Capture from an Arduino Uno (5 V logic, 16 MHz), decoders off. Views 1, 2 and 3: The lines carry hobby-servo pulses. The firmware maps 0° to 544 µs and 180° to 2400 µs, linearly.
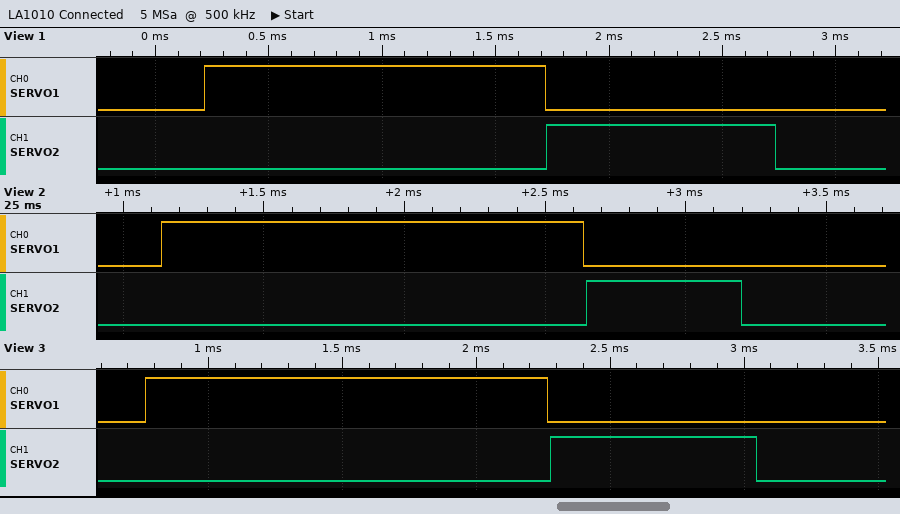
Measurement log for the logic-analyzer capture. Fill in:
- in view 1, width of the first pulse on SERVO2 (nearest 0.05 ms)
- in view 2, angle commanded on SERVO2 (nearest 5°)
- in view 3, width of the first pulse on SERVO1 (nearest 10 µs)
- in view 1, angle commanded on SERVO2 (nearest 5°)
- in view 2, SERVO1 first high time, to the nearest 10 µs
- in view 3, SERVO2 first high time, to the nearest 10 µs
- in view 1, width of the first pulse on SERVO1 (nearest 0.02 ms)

1.00 ms
0°
1500 µs
45°
1500 µs
770 µs
1.50 ms
